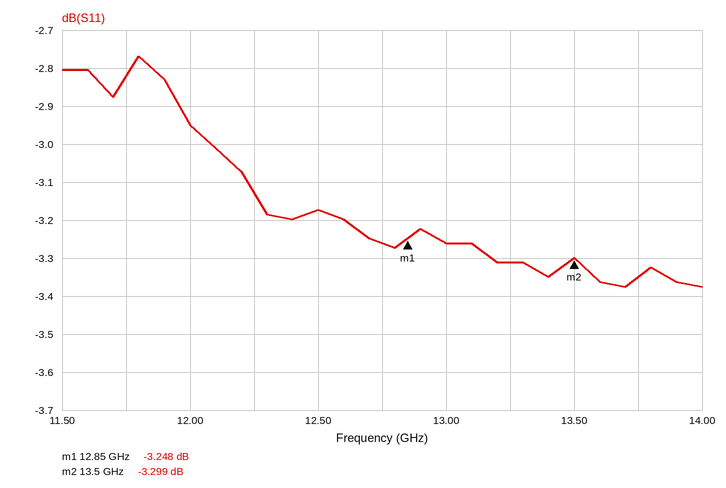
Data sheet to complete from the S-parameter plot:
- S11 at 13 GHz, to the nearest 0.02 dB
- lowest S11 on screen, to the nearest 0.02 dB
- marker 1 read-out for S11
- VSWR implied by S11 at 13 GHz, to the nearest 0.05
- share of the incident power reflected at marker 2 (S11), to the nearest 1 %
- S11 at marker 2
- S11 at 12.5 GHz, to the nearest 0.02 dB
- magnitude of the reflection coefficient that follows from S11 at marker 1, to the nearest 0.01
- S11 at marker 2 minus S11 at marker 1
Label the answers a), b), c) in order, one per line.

a) -3.26 dB
b) -3.38 dB
c) -3.248 dB
d) 5.40
e) 47 %
f) -3.299 dB
g) -3.18 dB
h) 0.69
i) -0.051 dB
